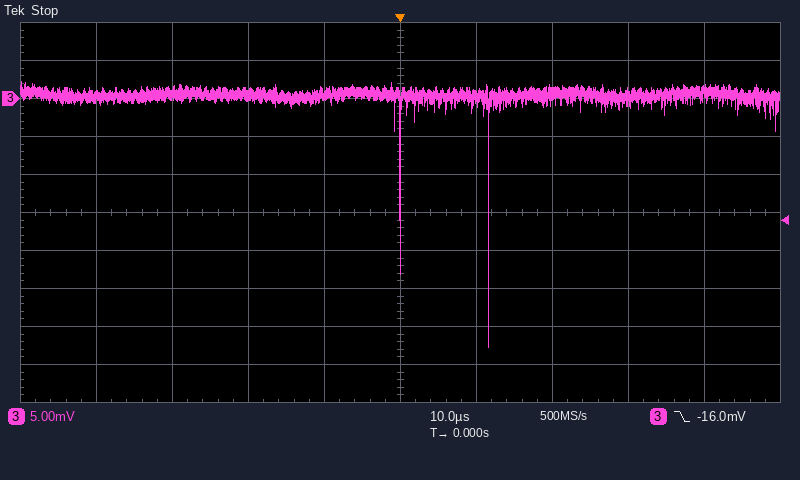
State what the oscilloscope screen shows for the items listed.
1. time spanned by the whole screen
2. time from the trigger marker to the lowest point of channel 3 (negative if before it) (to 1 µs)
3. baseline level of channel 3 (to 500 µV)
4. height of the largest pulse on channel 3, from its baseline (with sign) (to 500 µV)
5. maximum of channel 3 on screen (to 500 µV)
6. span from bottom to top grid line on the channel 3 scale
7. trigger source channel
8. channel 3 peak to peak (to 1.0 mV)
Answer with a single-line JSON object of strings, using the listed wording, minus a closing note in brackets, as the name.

{"time spanned by the whole screen": "100 µs", "time from the trigger marker to the lowest point of channel 3 (negative if before it)": "+12 µs", "baseline level of channel 3": "500 µV", "height of the largest pulse on channel 3, from its baseline (with sign)": "-33.0 mV", "maximum of channel 3 on screen": "2.0 mV", "span from bottom to top grid line on the channel 3 scale": "50 mV", "trigger source channel": "channel 3", "channel 3 peak to peak": "35.0 mV"}
